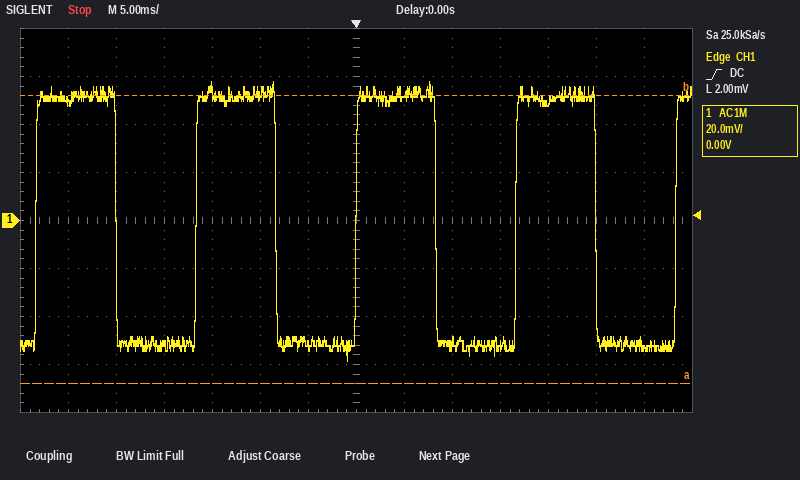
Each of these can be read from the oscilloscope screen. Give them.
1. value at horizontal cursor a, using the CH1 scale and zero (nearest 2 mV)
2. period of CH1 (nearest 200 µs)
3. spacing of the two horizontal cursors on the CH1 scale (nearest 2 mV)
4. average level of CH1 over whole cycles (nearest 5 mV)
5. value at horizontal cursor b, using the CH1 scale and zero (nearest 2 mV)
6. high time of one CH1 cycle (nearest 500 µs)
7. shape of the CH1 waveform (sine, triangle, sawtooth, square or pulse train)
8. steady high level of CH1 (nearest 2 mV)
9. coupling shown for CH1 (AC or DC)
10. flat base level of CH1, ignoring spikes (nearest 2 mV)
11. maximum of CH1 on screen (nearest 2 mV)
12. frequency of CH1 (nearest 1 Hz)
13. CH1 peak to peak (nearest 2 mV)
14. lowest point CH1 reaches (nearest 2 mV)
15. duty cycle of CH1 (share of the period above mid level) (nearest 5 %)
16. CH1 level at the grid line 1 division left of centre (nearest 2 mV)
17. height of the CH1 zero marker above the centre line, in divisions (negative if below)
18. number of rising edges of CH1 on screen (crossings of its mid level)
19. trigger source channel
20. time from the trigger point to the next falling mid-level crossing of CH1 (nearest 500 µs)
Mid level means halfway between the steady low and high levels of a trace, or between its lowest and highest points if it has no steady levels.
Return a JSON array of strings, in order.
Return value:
["-68 mV", "16.6 ms", "120 mV", "0 mV", "52 mV", "8.5 ms", "square", "52 mV", "AC", "-52 mV", "58 mV", "60 Hz", "116 mV", "-58 mV", "50 %", "-52 mV", "0.0 div", "5", "CH1", "8.5 ms"]
